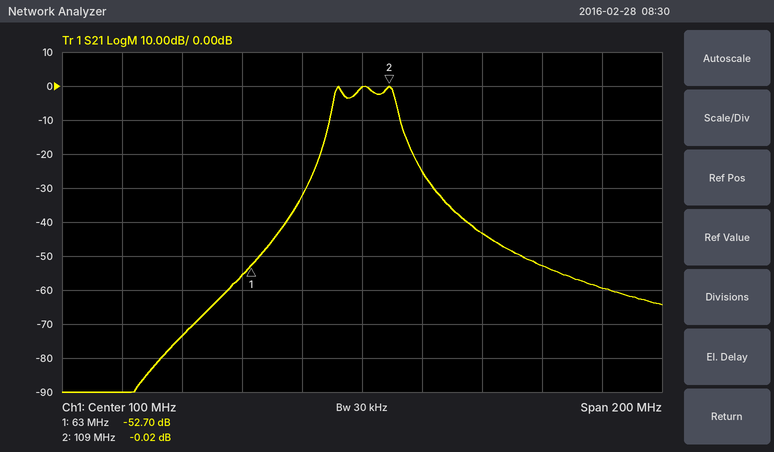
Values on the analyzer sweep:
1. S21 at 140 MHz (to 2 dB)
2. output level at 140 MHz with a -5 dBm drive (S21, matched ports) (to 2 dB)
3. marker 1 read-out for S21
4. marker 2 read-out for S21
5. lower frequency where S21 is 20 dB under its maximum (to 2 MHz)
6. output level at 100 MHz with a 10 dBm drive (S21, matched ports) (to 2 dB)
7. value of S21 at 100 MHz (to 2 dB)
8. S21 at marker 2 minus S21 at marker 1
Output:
-44 dB
-48 dBm
-52.70 dB
-0.02 dB
86 MHz
10 dBm
0 dB
52.68 dB
